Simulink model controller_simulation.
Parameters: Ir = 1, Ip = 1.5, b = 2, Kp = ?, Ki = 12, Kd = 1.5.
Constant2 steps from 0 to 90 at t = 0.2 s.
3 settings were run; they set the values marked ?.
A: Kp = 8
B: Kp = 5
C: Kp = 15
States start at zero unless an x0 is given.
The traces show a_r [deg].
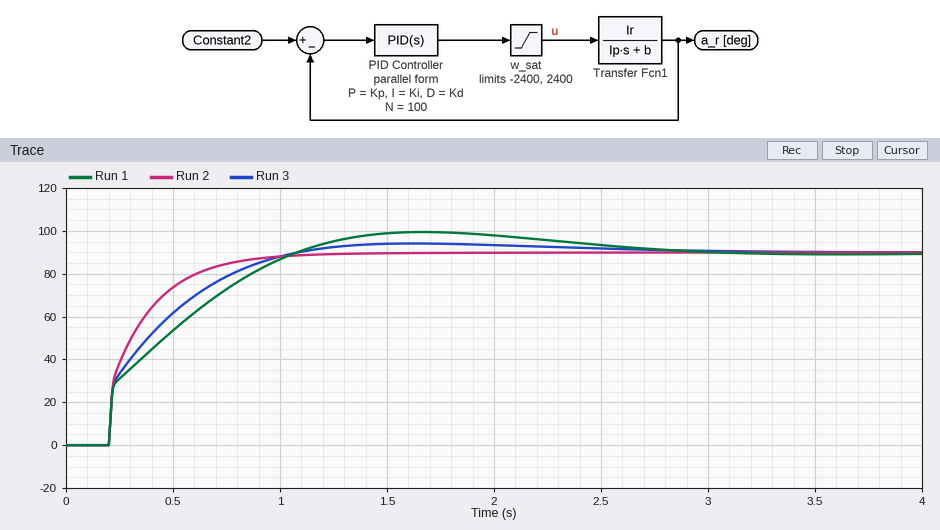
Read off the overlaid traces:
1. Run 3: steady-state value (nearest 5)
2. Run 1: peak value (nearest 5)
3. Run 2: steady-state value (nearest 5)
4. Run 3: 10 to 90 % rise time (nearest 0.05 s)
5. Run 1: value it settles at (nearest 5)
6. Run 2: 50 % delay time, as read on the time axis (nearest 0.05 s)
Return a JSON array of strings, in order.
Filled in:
["90", "100", "90", "0.60 s", "90", "0.30 s"]
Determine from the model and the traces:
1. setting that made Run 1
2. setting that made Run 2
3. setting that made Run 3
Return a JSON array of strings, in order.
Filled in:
["B", "C", "A"]
